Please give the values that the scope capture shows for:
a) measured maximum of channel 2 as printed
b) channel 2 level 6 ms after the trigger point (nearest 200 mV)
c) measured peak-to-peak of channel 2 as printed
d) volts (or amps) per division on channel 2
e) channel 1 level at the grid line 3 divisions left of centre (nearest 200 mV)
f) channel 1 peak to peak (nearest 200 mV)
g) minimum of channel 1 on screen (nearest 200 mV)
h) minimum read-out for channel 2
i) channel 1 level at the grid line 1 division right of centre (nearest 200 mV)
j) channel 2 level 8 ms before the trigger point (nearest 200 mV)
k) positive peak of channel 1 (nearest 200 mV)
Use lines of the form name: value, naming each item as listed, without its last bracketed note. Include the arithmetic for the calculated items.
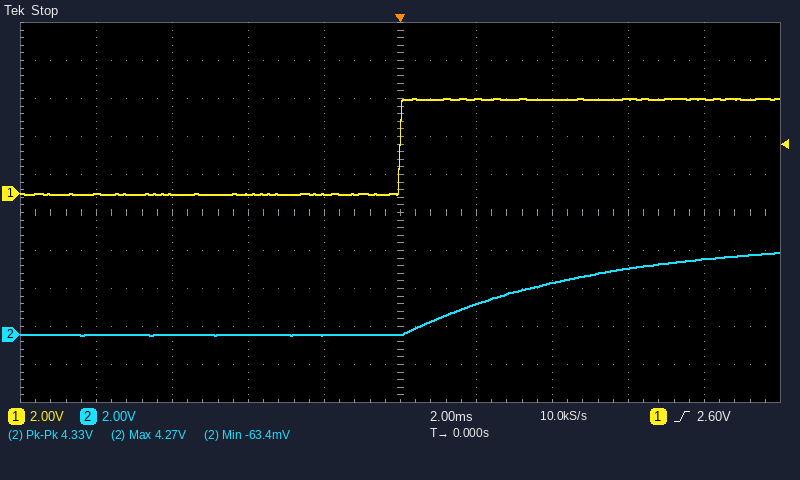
measured maximum of channel 2 as printed: 4.27 V
channel 2 level 6 ms after the trigger point: 3.4 V
measured peak-to-peak of channel 2 as printed: 4.33 V
volts (or amps) per division on channel 2: 2 V
channel 1 level at the grid line 3 divisions left of centre: 0.0 V
channel 1 peak to peak: 5.0 V − (0.0 V) = 5.0 V
minimum of channel 1 on screen: 0.0 V
minimum read-out for channel 2: -63.4 mV
channel 1 level at the grid line 1 division right of centre: 5.0 V
channel 2 level 8 ms before the trigger point: 0.0 V
positive peak of channel 1: 5.0 V
